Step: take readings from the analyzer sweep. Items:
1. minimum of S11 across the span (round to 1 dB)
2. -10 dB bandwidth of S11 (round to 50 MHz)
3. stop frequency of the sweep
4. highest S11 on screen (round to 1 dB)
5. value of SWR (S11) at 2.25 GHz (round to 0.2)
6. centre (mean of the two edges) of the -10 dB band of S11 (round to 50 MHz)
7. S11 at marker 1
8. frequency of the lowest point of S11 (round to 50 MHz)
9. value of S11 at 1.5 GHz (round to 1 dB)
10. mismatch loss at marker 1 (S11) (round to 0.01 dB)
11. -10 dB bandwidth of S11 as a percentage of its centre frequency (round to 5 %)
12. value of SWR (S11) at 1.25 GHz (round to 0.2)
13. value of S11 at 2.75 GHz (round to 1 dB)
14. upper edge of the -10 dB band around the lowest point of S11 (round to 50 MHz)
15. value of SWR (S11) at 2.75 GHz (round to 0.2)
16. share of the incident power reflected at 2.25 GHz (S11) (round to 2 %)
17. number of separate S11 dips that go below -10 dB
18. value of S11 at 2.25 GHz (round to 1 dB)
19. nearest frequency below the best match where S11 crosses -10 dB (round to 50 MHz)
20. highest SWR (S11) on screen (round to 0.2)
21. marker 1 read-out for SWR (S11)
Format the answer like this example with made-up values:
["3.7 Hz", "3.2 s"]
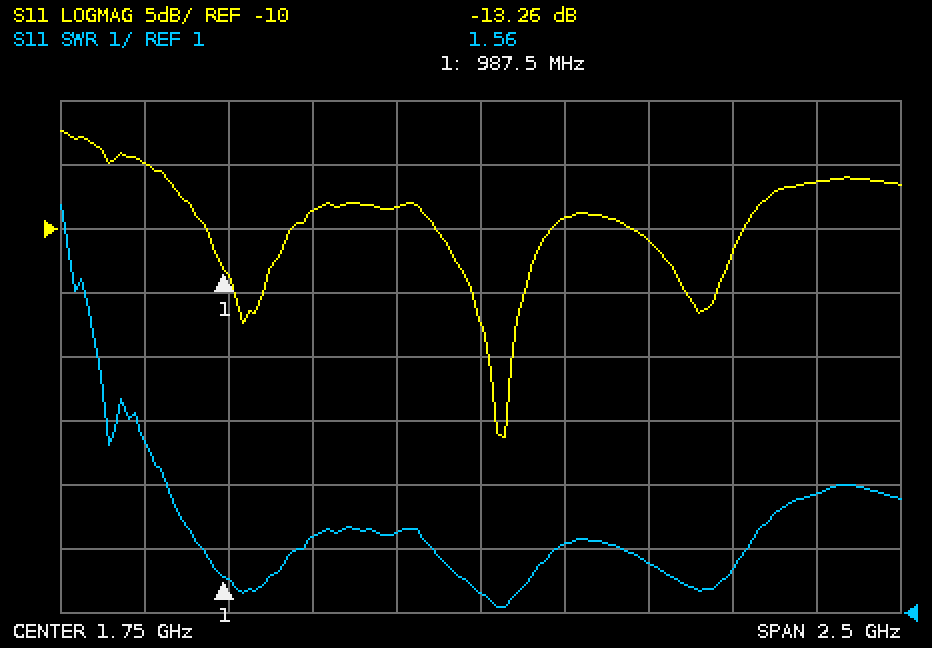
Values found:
["-26 dB", "350 MHz", "3 GHz", "-2 dB", "1.8", "1.80 GHz", "-13.26 dB", "1.80 GHz", "-8 dB", "0.21 dB", "20 %", "2.2", "-6 dB", "1.95 GHz", "2.8", "8 %", "3", "-11 dB", "1.60 GHz", "7.4", "1.56"]
